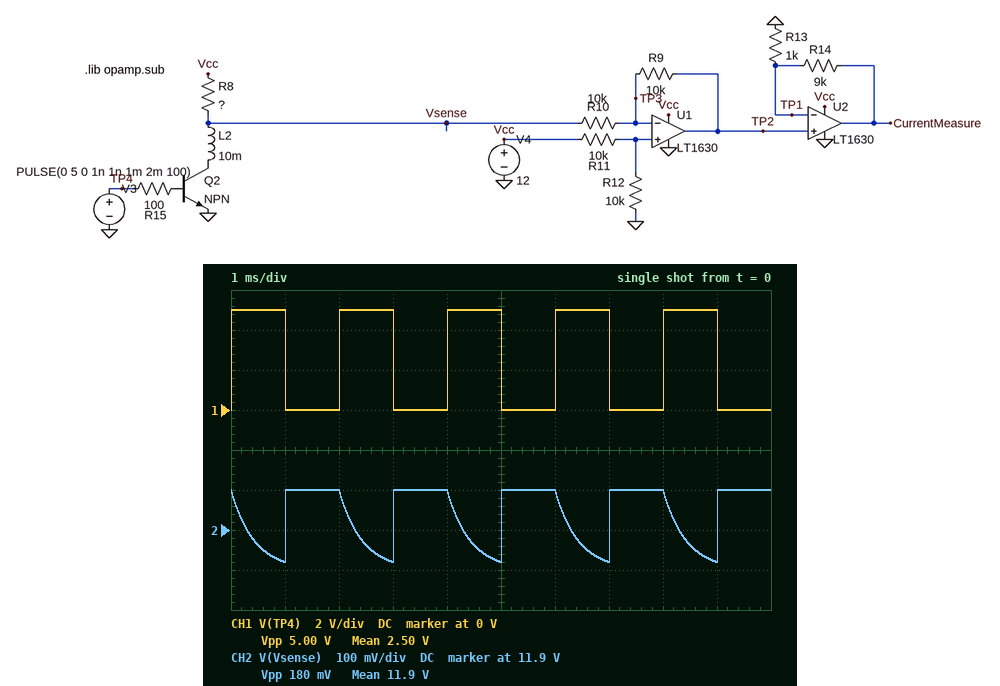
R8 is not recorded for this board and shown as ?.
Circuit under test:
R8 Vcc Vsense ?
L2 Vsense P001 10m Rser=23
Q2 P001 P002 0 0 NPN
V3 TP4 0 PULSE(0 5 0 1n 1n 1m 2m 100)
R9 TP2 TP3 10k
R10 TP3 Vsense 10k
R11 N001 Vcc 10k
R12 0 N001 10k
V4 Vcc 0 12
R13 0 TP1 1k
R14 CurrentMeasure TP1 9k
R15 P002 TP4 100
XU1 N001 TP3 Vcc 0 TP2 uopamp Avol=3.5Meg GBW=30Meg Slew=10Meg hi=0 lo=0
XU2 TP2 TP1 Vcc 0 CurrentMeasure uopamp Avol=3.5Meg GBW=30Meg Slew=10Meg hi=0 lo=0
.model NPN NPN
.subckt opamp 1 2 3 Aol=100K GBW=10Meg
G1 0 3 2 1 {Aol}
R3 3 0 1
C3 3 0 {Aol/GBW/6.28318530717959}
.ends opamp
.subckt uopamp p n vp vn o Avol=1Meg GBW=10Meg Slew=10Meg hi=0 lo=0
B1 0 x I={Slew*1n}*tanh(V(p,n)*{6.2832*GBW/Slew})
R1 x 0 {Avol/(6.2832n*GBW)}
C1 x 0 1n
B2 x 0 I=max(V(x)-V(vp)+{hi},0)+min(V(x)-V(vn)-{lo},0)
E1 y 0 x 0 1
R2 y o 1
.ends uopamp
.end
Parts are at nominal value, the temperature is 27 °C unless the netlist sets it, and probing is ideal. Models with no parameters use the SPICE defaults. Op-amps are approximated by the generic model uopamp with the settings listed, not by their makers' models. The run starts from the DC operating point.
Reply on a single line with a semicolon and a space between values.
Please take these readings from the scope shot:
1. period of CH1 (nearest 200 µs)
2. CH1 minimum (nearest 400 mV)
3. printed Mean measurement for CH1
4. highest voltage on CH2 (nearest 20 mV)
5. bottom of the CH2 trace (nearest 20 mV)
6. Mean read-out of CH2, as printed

2.0 ms; 0 V; 2.50 V; 12.00 V; 11.82 V; 11.9 V
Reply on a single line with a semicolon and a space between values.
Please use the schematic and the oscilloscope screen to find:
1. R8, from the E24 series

0.39 Ω
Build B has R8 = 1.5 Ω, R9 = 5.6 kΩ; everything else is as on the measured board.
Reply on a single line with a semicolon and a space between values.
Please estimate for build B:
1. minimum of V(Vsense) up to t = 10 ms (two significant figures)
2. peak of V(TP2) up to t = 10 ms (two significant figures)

11 V; 3.0 V
